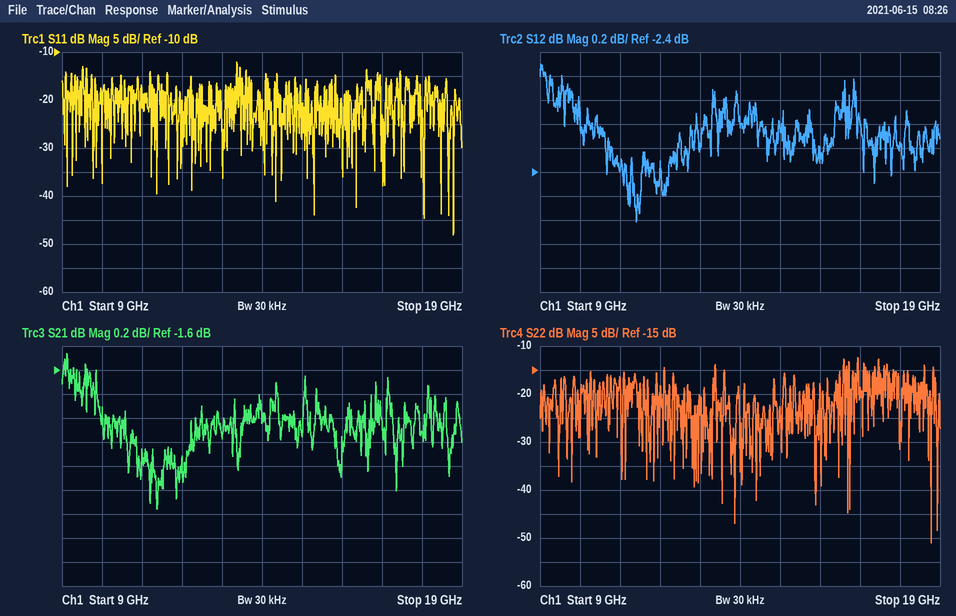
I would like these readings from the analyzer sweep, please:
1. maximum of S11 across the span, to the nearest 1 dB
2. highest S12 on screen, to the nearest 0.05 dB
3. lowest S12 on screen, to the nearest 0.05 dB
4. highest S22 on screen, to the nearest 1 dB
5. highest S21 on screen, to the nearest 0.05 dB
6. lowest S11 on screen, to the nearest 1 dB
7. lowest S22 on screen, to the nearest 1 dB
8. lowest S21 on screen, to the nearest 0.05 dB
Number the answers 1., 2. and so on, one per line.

1. -12 dB
2. -1.50 dB
3. -2.80 dB
4. -12 dB
5. -1.45 dB
6. -48 dB
7. -51 dB
8. -2.75 dB
